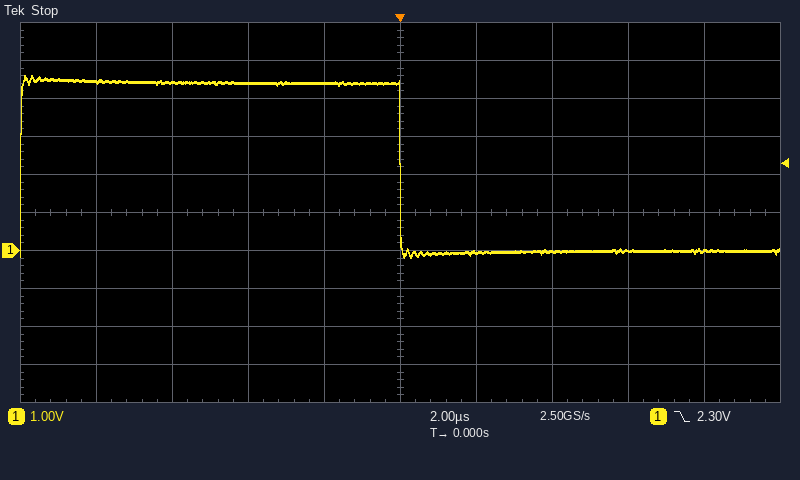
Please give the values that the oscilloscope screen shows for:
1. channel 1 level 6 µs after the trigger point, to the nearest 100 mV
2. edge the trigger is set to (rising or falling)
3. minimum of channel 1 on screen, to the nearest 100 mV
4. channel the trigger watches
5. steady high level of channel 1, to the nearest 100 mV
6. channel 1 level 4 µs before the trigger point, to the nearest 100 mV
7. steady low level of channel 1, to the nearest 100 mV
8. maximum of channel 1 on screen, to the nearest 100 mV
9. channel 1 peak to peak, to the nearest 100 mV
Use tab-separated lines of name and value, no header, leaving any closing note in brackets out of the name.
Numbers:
channel 1 level 6 µs after the trigger point, to the nearest 100 mV	0.0 V
edge the trigger is set to	falling
minimum of channel 1 on screen, to the nearest 100 mV	-200 mV
channel the trigger watches	channel 1
steady high level of channel 1, to the nearest 100 mV	4.4 V
channel 1 level 4 µs before the trigger point, to the nearest 100 mV	4.4 V
steady low level of channel 1, to the nearest 100 mV	0.0 V
maximum of channel 1 on screen, to the nearest 100 mV	4.6 V
channel 1 peak to peak, to the nearest 100 mV	4.8 V
